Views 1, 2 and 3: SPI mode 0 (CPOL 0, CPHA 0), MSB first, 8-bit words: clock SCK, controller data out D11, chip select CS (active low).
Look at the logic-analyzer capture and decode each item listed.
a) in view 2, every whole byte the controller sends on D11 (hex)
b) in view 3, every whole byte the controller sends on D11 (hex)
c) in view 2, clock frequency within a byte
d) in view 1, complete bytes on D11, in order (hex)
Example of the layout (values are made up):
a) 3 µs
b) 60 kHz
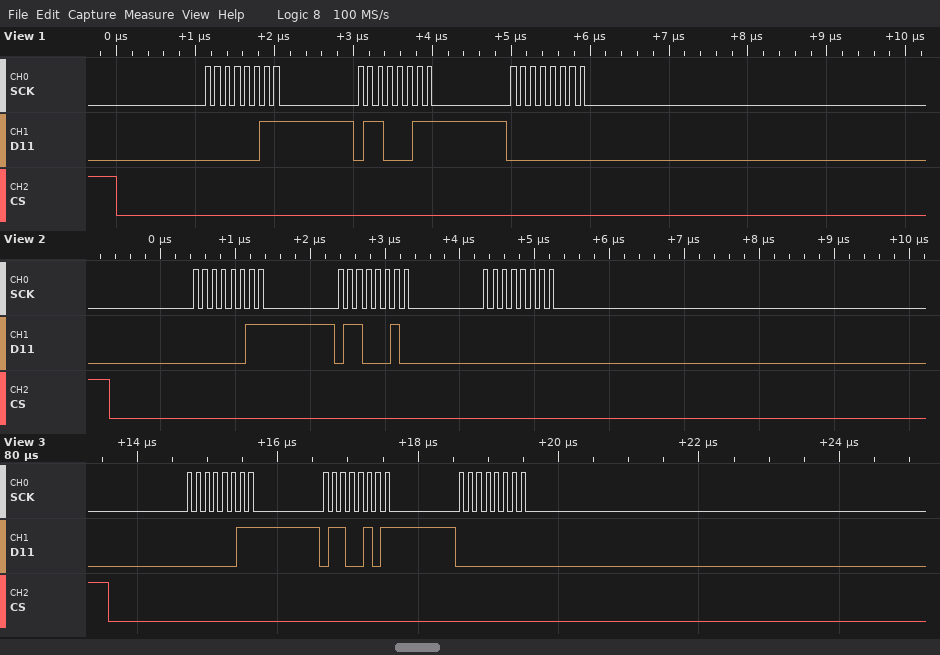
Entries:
a) 03 62 00
b) 03 65 00
c) 8 MHz
d) 03 63 00
